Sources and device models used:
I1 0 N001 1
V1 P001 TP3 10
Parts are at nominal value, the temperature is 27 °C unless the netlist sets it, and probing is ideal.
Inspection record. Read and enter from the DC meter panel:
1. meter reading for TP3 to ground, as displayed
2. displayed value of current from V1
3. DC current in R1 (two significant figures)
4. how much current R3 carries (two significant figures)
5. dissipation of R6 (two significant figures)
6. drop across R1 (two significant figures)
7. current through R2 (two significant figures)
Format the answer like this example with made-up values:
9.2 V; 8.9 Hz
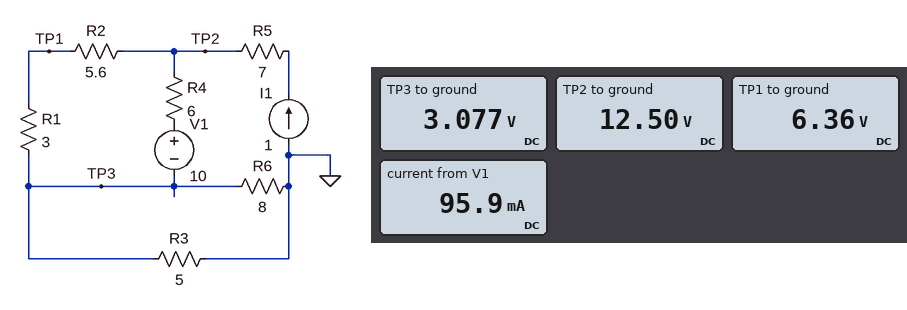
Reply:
3.077 V; 95.9 mA; 1.1 A; 620 mA; 1.2 W; 3.3 V; 1.1 A
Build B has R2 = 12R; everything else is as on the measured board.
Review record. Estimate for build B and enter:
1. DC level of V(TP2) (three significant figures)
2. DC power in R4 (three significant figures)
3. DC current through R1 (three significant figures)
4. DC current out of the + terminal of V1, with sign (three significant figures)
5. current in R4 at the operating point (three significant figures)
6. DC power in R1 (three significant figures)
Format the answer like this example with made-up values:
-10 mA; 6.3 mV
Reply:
14.5 V; 340 mW; 762 mA; -238 mA; 238 mA; 1.74 W
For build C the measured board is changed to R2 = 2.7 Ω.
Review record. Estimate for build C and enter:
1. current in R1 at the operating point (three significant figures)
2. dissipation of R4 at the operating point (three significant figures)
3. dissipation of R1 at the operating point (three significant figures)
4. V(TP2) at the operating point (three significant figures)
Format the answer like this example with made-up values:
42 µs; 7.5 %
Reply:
1.37 A; 810 mW; 5.61 W; 10.9 V
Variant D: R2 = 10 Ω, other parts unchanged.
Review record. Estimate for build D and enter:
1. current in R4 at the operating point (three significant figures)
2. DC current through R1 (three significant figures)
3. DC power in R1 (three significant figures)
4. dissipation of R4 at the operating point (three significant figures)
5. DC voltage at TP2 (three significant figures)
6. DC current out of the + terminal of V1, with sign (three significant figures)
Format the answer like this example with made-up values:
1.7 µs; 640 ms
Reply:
158 mA; 842 mA; 2.13 W; 150 mW; 14.0 V; -158 mA
